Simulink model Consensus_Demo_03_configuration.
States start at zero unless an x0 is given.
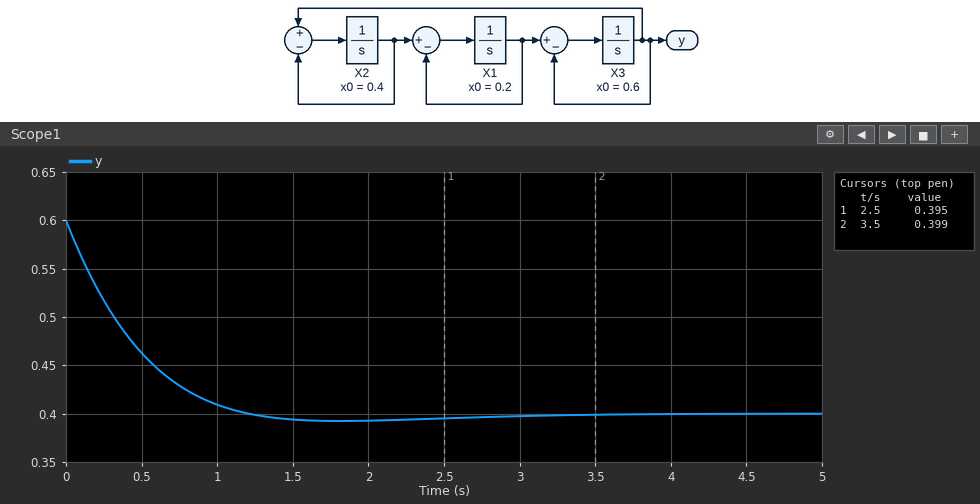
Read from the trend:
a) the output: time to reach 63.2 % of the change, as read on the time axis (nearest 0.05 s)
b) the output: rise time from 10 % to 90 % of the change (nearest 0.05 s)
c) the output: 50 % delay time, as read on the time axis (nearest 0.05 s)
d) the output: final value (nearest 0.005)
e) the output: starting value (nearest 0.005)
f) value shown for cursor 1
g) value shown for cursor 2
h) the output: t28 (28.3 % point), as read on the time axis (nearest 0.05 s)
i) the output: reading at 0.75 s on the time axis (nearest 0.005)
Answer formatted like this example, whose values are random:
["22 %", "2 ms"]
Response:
["0.45 s", "0.80 s", "0.30 s", "0.400", "0.600", "0.395", "0.399", "0.15 s", "0.430"]
